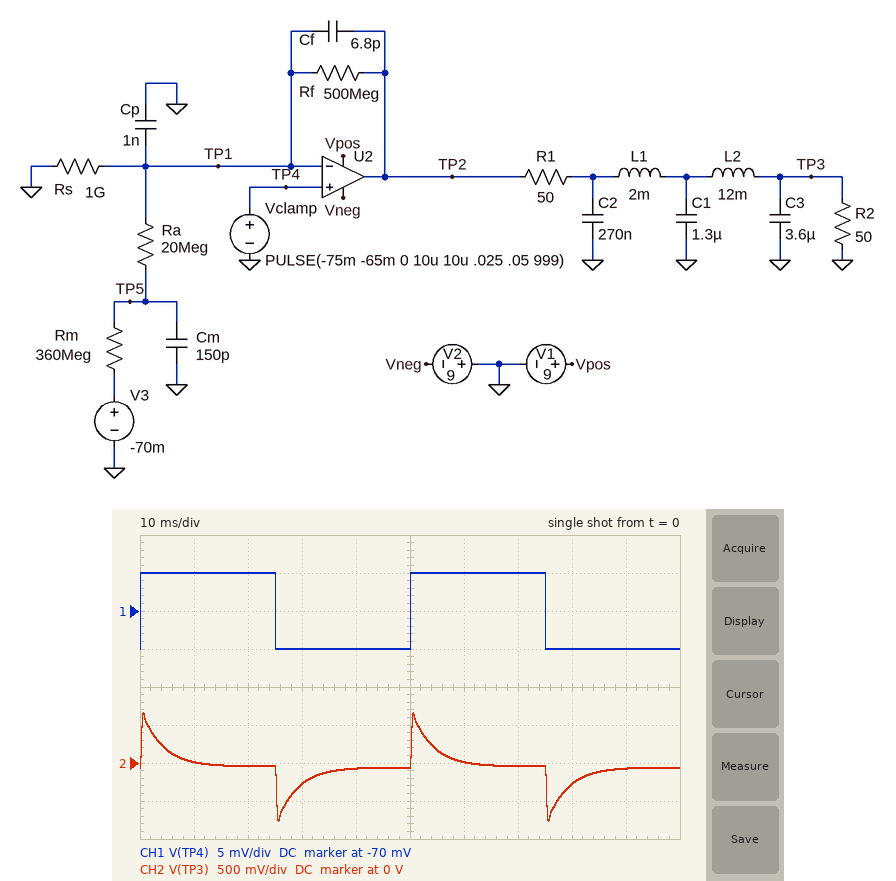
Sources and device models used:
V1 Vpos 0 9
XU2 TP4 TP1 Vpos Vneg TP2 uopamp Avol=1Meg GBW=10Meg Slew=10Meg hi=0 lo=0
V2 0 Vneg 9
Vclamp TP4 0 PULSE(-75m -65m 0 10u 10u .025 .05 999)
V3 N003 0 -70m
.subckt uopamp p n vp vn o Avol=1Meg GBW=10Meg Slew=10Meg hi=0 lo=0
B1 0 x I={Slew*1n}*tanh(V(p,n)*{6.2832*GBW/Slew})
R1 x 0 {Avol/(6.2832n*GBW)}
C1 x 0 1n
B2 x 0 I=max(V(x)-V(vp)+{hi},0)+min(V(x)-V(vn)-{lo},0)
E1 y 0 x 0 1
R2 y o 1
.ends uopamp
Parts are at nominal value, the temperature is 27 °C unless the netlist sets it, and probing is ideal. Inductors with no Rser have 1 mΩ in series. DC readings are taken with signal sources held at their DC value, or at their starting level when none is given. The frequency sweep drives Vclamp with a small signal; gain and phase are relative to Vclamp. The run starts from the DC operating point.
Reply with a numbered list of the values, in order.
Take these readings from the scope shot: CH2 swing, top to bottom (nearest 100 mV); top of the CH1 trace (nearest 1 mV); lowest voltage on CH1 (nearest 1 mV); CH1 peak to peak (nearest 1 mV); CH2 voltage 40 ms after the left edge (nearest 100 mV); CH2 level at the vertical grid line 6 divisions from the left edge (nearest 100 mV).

1. 1.4 V
2. -65 mV
3. -75 mV
4. 10 mV
5. -100 mV
6. 0 V
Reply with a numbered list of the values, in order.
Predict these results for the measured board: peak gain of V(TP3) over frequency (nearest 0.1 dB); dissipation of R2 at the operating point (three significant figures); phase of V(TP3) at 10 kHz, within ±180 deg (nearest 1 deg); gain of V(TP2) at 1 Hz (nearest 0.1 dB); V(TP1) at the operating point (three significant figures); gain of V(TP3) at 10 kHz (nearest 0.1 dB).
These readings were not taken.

1. 37.3 dB
2. 70.9 µW
3. -25 deg
4. 13.2 dB
5. -75.0 mV
6. -21.1 dB
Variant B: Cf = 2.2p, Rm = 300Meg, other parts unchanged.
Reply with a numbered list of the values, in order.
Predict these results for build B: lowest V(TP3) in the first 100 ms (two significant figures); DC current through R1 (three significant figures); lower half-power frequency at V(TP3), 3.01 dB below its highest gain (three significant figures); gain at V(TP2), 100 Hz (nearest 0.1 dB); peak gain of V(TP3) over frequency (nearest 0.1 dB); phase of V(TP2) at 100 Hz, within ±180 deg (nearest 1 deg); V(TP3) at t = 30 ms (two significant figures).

1. -1.9 V
2. 1.20 mA
3. 126 Hz
4. 48.6 dB
5. 46.7 dB
6. 52 deg
7. -120 mV
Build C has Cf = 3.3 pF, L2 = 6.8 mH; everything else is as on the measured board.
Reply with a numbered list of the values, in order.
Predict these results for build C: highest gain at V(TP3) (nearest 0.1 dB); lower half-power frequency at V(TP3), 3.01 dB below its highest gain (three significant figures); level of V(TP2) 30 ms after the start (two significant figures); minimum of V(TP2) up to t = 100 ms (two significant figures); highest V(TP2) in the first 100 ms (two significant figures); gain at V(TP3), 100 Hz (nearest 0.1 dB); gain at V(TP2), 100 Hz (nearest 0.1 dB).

1. 43.4 dB
2. 84.8 Hz
3. -340 mV
4. -3.1 V
5. 2.9 V
6. 41.1 dB
7. 47.1 dB
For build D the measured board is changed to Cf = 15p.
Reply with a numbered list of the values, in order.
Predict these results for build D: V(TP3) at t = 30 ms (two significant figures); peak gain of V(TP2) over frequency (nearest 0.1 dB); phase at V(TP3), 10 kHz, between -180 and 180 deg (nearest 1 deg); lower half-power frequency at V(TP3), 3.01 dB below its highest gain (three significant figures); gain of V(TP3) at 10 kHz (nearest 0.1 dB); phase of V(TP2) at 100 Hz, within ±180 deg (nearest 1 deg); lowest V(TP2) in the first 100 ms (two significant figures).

1. -250 mV
2. 36.7 dB
3. -21 deg
4. 17.5 Hz
5. -27.9 dB
6. 8 deg
7. -740 mV
